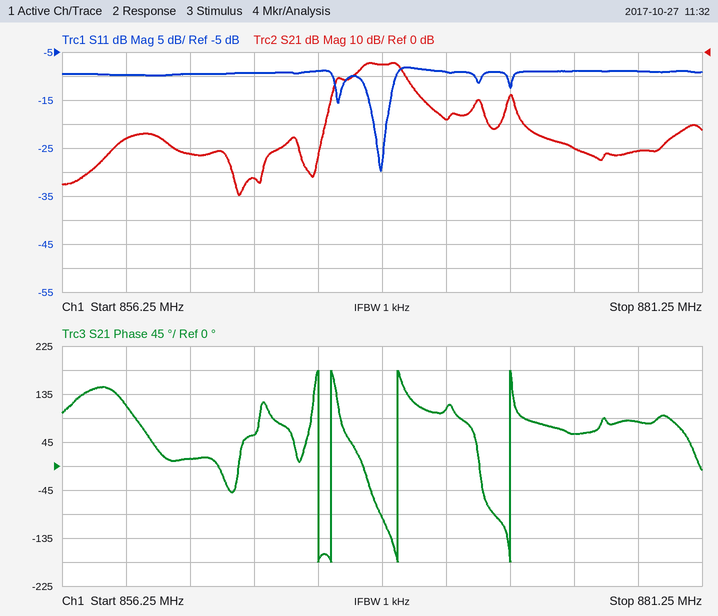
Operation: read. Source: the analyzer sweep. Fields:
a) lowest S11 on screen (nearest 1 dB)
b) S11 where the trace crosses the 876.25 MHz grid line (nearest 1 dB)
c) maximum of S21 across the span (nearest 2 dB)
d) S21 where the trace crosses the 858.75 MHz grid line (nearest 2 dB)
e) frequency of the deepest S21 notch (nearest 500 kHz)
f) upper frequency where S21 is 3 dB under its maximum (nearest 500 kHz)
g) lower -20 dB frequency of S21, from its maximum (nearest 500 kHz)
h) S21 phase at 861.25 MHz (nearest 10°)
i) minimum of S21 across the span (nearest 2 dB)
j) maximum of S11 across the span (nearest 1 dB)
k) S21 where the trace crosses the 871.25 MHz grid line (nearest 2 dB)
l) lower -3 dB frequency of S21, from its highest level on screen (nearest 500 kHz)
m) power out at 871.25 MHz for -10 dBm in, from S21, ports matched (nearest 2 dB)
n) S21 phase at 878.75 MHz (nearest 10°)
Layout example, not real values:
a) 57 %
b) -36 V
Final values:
a) -30 dB
b) -9 dB
c) -4 dB
d) -36 dB
e) 863.0 MHz
f) 869.5 MHz
g) 866.5 MHz
h) 10°
i) -60 dB
j) -8 dB
k) -28 dB
l) 868.0 MHz
m) -38 dBm
n) 80°
